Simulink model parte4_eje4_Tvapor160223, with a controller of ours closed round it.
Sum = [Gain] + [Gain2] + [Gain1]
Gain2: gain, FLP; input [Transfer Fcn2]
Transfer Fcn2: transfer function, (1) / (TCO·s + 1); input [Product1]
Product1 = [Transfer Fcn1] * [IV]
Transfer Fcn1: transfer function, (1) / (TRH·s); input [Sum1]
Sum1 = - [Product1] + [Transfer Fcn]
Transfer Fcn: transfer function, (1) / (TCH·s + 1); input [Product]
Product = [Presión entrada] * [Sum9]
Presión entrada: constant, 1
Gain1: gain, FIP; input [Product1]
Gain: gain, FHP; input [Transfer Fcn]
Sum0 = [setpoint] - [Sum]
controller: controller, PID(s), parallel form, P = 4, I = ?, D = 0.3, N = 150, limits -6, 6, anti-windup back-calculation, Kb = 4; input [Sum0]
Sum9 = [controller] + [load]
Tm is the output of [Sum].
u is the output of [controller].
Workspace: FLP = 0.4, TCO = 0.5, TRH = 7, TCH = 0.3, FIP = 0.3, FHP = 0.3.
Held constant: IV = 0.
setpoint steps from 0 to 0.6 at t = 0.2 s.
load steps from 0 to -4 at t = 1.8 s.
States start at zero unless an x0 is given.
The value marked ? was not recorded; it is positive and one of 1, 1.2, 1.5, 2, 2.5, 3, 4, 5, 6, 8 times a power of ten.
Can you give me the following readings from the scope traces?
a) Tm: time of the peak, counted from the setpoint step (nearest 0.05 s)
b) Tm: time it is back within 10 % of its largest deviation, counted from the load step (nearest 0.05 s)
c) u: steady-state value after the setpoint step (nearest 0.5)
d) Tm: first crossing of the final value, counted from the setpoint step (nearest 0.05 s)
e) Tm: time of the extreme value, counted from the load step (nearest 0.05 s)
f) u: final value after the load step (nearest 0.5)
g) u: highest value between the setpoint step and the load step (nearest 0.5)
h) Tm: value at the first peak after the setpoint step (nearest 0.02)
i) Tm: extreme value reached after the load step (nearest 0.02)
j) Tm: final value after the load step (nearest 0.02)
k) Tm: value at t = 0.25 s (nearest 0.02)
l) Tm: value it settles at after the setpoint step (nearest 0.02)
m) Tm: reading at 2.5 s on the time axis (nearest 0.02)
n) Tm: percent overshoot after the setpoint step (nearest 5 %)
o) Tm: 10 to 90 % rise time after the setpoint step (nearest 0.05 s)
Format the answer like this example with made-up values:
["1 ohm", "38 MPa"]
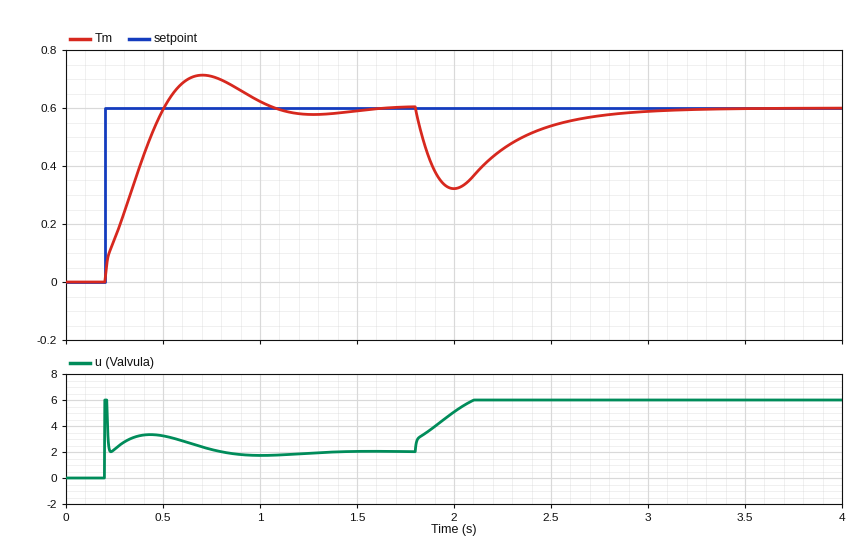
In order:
["0.50 s", "0.95 s", "2.0", "0.30 s", "0.20 s", "6.0", "6.0", "0.72", "0.32", "0.60", "0.14", "0.60", "0.54", "20 %", "0.25 s"]
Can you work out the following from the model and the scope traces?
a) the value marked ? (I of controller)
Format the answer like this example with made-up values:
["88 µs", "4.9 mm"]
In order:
["50"]
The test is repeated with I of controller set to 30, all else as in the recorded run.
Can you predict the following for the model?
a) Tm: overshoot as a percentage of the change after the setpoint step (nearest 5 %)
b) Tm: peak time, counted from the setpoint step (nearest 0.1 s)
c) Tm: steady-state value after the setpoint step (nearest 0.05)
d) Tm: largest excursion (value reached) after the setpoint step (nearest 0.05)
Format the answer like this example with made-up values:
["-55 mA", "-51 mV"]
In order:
["10 %", "0.7 s", "0.60", "0.65"]
